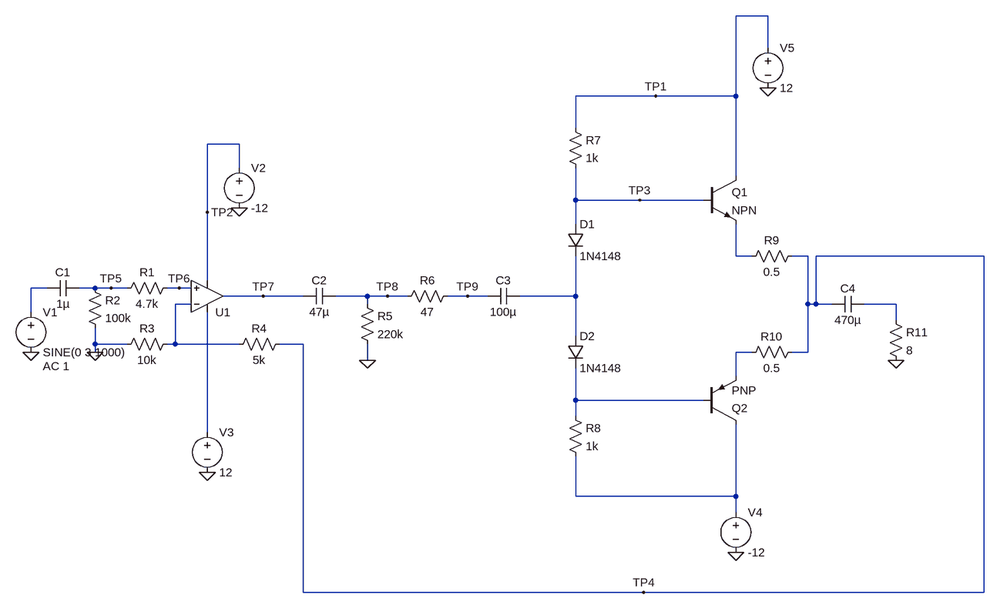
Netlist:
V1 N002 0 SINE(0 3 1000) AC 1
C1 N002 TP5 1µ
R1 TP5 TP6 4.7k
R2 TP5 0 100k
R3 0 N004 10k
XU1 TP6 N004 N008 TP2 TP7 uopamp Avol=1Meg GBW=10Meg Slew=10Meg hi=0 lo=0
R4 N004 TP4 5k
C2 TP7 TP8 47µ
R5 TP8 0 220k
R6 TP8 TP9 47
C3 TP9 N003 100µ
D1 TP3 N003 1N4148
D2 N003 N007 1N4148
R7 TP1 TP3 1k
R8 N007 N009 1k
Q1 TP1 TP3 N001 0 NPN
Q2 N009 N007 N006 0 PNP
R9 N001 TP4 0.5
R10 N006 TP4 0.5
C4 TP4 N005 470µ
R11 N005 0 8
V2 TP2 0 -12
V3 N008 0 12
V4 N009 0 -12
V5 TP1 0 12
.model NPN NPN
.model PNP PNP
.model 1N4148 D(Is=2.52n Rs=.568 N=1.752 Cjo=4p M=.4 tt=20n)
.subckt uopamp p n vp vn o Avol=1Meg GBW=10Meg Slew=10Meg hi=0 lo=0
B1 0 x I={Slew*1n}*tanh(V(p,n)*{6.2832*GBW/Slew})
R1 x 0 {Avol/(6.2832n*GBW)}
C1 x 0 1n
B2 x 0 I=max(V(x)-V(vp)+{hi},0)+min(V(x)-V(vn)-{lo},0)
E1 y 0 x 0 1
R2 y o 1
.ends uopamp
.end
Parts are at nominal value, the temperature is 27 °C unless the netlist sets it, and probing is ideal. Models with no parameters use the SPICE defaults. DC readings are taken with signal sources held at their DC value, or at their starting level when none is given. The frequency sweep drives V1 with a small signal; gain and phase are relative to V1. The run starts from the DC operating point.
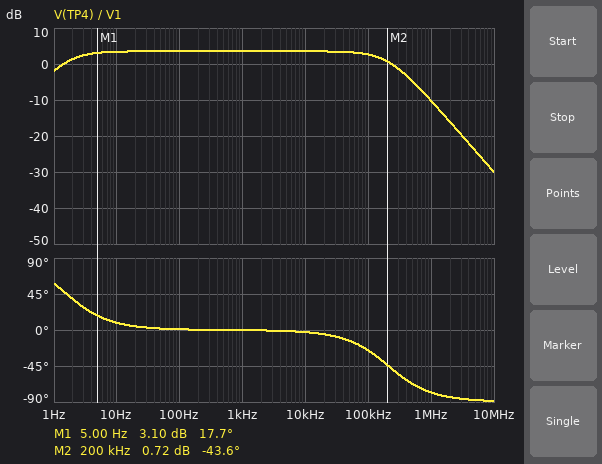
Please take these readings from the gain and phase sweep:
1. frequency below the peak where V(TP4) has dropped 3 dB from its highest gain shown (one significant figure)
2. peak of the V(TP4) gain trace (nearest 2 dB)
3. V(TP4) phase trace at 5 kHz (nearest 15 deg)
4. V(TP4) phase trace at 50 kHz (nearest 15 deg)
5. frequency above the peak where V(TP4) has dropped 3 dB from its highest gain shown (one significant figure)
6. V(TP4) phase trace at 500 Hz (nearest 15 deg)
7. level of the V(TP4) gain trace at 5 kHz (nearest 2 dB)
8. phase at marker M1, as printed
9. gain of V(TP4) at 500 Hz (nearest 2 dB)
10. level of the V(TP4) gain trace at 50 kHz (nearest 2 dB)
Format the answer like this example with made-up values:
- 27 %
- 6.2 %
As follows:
- 2 Hz
- 4 dB
- 0 deg
- -15 deg
- 200 kHz
- 0 deg
- 4 dB
- 17.7 deg
- 4 dB
- 4 dB
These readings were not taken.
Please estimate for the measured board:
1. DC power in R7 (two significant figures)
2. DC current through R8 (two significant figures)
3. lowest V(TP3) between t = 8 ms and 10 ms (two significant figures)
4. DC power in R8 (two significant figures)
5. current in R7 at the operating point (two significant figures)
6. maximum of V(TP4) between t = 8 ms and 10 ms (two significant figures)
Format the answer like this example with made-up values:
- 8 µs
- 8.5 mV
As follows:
- 130 mW
- 11 mA
- -4.4 V
- 130 mW
- 11 mA
- 4.5 V
